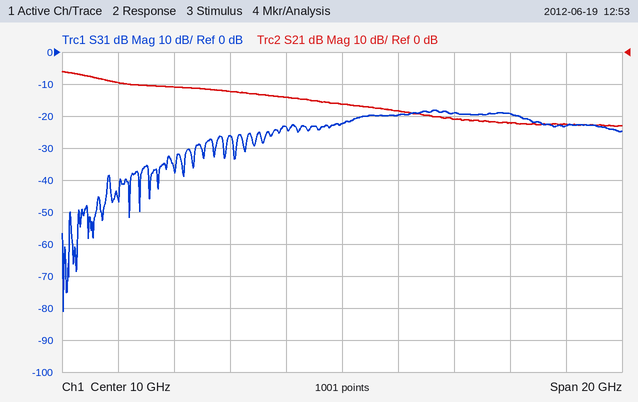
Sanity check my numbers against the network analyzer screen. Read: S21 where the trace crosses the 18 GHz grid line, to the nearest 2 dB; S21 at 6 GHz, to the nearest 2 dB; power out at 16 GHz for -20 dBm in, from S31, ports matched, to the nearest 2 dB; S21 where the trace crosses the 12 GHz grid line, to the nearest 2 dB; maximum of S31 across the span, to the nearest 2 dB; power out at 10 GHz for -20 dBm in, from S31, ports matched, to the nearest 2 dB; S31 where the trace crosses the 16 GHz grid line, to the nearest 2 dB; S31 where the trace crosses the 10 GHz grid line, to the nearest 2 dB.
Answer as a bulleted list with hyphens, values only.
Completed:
- -22 dB
- -12 dB
- -40 dBm
- -18 dB
- -18 dB
- -42 dBm
- -20 dB
- -22 dB
